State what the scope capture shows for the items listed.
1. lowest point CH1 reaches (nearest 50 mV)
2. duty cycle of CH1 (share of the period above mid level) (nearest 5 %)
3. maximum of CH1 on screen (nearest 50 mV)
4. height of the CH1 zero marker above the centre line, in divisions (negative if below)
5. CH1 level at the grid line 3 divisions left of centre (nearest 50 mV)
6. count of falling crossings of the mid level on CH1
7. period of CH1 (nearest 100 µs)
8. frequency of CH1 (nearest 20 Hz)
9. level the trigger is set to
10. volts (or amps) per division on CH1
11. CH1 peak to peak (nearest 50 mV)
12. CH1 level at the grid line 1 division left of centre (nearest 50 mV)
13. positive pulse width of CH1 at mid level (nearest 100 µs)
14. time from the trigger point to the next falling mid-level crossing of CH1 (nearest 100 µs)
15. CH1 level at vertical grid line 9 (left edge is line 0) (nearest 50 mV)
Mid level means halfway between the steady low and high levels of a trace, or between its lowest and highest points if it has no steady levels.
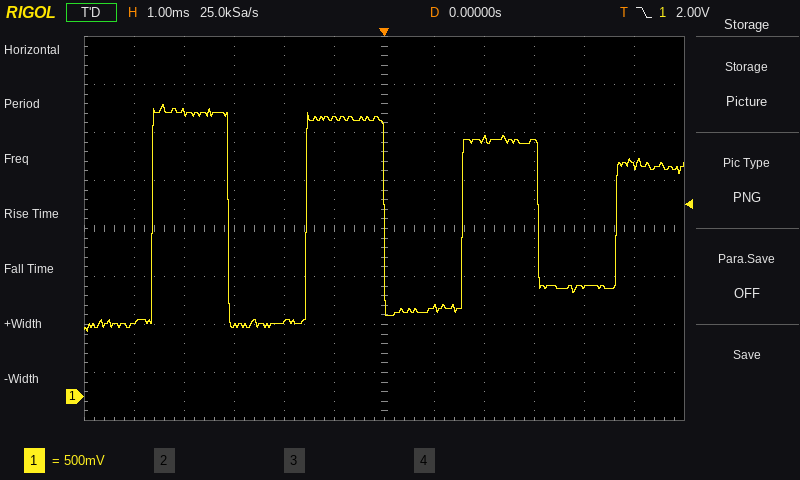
700 mV
50 %
3.05 V
-3.5 div
750 mV
3
3.1 ms
320 Hz
2.00 V
500 mV
2.35 V
2.90 V
1.5 ms
3.1 ms
2.65 V
